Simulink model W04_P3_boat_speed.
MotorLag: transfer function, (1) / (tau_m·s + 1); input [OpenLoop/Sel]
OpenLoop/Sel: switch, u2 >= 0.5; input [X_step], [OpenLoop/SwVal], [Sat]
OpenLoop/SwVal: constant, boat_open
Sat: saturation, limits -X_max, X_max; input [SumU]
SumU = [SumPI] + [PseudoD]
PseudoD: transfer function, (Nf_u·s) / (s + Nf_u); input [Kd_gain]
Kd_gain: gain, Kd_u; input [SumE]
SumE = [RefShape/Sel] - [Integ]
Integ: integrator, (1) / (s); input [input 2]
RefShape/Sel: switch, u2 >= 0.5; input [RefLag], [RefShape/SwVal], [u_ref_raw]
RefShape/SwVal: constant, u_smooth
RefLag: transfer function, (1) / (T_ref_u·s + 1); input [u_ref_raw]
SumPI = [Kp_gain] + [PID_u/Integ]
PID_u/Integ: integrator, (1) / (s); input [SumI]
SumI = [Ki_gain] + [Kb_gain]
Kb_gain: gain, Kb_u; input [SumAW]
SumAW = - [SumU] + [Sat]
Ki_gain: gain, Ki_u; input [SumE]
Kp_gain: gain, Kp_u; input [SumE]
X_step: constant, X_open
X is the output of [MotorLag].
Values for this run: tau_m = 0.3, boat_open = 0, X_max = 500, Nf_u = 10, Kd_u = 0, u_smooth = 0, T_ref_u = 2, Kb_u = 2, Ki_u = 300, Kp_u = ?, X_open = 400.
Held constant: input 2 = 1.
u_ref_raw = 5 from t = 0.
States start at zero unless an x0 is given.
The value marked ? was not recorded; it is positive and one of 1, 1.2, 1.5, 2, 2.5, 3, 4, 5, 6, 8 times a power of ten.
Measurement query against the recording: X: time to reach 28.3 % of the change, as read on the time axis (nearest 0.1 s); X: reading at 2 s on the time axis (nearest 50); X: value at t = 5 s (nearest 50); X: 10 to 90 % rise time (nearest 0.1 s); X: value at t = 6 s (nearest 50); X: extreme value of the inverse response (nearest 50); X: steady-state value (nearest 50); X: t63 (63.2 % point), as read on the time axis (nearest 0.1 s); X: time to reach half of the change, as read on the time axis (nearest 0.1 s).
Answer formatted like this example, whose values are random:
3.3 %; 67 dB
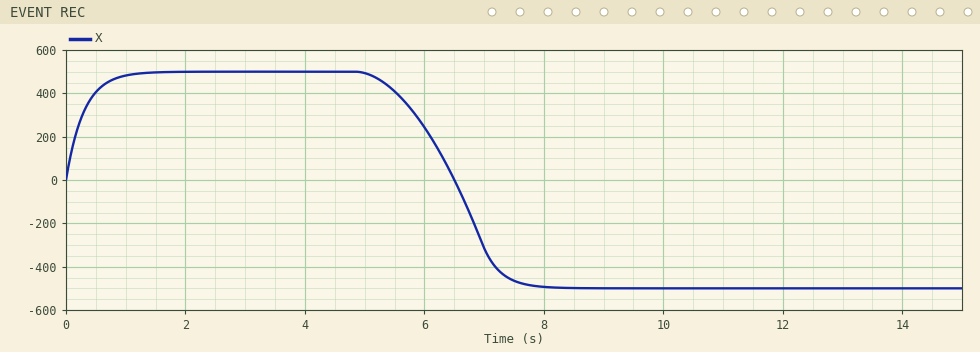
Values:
6.7 s; 500; 500; 0.8 s; 250; 500; -500; 7.0 s; 6.9 s
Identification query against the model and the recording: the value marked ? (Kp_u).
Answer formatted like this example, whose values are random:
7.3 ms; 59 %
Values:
200
